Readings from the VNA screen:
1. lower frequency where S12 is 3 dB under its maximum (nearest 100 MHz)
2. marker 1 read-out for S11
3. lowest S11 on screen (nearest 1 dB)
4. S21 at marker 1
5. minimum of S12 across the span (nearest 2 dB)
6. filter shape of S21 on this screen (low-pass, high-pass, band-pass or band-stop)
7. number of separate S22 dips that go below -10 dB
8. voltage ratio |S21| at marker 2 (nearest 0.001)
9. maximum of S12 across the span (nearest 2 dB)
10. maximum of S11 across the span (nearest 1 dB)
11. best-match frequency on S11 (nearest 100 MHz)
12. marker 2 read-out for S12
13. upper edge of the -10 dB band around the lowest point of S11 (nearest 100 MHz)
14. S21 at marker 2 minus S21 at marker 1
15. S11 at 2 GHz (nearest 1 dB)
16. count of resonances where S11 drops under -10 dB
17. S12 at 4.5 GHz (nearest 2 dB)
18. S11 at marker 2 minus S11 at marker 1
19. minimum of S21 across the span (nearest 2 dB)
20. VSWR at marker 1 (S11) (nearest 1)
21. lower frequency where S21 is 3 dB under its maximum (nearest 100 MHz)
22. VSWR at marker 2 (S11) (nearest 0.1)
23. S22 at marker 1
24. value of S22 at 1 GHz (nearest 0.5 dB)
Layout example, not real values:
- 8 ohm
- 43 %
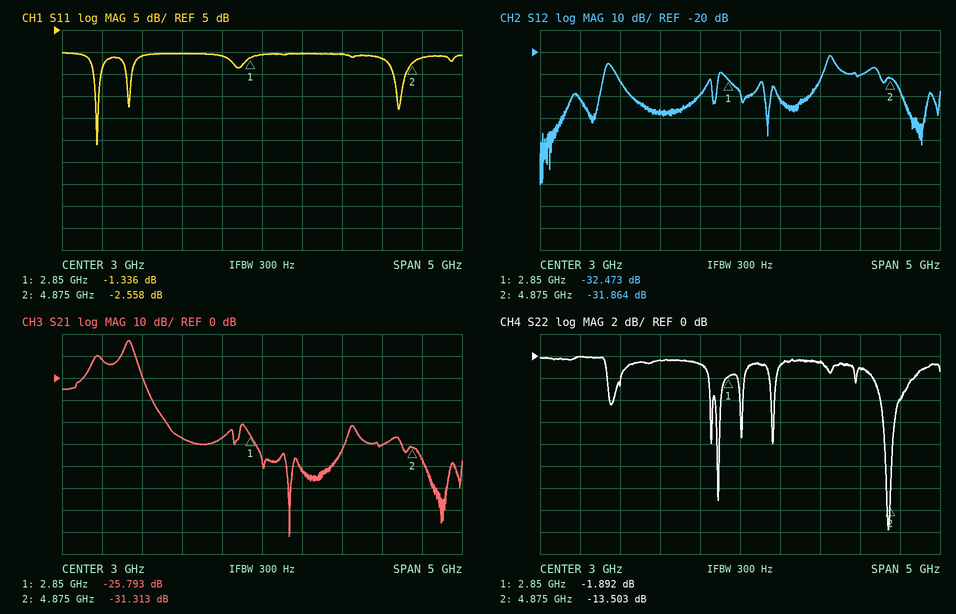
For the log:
- 4.1 GHz
- -1.336 dB
- -21 dB
- -25.793 dB
- -80 dB
- band-pass
- 2
- 0.027
- -22 dB
- 0 dB
- 900 MHz
- -31.864 dB
- 1.0 GHz
- -5.520 dB
- 0 dB
- 3
- -30 dB
- -1.222 dB
- -72 dB
- 13
- 1.3 GHz
- 6.8
- -1.892 dB
- 0.0 dB
